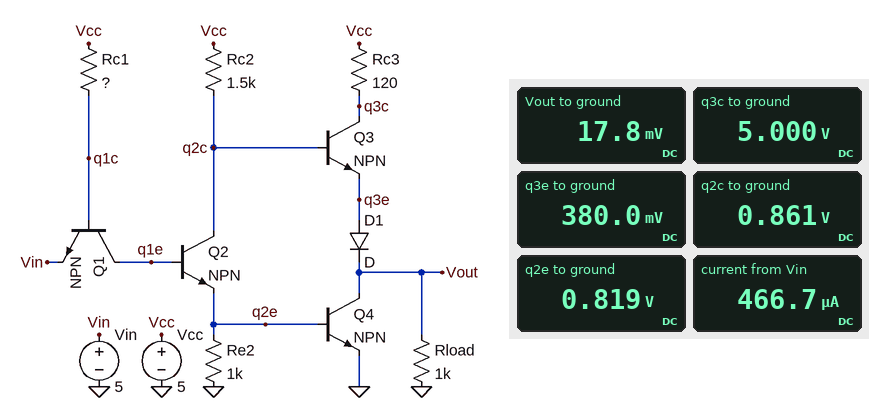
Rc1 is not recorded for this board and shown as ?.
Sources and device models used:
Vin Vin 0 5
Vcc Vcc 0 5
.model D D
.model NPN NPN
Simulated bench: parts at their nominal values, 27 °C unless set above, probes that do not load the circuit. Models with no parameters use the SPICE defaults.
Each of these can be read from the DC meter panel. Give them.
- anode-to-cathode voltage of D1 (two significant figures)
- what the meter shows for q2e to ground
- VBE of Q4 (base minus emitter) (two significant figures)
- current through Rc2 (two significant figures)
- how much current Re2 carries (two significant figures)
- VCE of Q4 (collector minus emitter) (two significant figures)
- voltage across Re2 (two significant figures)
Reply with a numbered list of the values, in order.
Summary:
1. 360 mV
2. 0.819 V
3. 820 mV
4. 2.8 mA
5. 820 µA
6. 18 mV
7. 820 mV
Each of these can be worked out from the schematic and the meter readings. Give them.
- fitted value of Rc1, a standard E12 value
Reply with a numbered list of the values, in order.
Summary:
1. 5.6 kΩ
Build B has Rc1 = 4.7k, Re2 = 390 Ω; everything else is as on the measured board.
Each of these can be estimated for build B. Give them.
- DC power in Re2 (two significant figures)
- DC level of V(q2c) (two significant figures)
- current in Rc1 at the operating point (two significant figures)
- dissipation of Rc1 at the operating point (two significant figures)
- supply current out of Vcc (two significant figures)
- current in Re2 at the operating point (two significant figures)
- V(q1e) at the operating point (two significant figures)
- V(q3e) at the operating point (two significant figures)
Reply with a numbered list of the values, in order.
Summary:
1. 1.7 mW
2. 850 mV
3. 560 µA
4. 1.5 mW
5. 3.3 mA
6. 2.1 mA
7. 1.6 V
8. 370 mV
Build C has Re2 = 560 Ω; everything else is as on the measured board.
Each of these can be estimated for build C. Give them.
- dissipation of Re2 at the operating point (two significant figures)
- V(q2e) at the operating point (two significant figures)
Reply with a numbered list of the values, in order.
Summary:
1. 1.2 mW
2. 810 mV
